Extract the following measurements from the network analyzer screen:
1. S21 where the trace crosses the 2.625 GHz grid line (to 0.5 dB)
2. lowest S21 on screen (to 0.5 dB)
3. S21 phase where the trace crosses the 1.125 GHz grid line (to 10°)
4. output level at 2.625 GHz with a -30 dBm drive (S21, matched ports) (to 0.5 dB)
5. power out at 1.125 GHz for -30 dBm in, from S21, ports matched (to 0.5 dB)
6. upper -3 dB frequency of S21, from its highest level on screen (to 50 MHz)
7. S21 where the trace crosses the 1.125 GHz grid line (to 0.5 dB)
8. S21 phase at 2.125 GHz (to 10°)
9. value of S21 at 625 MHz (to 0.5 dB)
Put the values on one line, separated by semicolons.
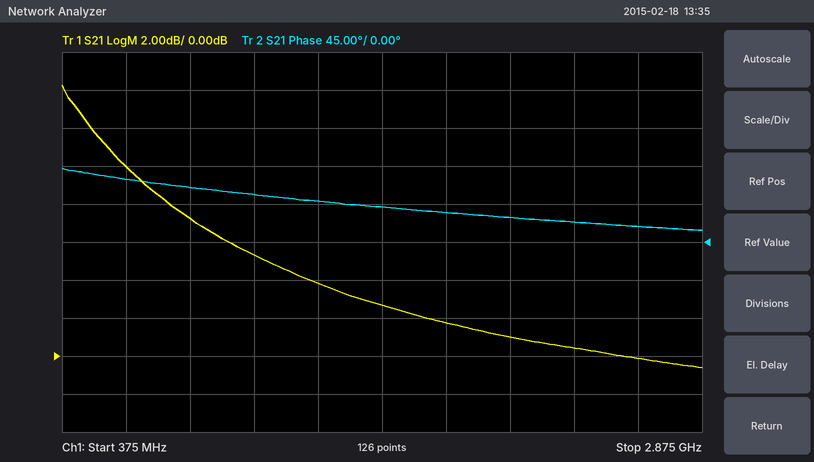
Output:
0.0 dB; -0.5 dB; 60°; -30.0 dBm; -24.5 dBm; 550 MHz; 5.5 dB; 30°; 10.0 dB
